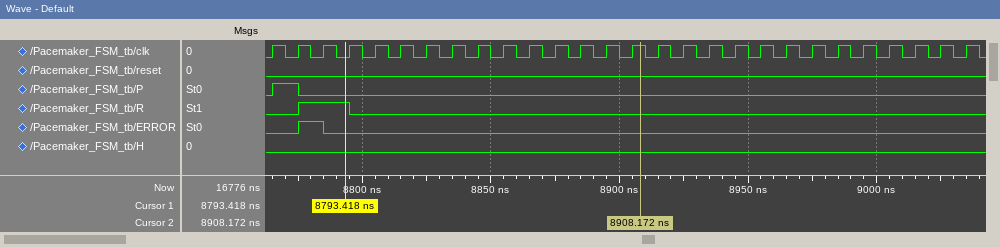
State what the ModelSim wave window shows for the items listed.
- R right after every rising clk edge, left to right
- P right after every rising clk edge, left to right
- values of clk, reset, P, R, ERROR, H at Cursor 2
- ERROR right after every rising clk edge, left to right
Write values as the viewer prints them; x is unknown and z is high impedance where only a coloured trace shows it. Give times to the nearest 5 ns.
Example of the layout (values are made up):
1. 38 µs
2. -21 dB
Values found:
1. 0 1 1 0 0 0 0 0 0 0 0 0 0 0 0 0 0 0 0 0 0 0 0 0 0 0 0 0
2. 1 0 0 0 0 0 0 0 0 0 0 0 0 0 0 0 0 0 0 0 0 0 0 0 0 0 0 0
3. clk=1, reset=0, P=0, R=0, ERROR=0, H=0
4. 0 1 0 0 0 0 0 0 0 0 0 0 0 0 0 0 0 0 0 0 0 0 0 0 0 0 0 0
